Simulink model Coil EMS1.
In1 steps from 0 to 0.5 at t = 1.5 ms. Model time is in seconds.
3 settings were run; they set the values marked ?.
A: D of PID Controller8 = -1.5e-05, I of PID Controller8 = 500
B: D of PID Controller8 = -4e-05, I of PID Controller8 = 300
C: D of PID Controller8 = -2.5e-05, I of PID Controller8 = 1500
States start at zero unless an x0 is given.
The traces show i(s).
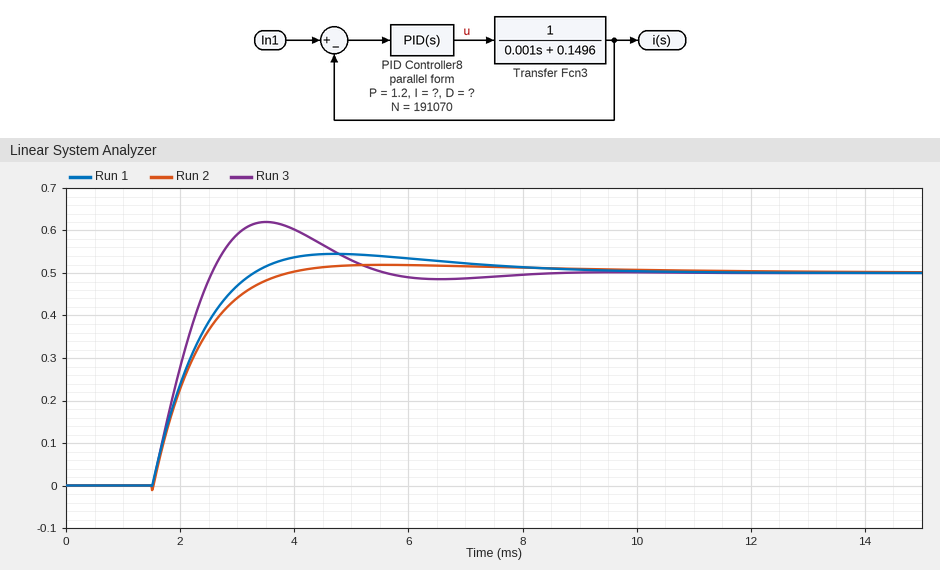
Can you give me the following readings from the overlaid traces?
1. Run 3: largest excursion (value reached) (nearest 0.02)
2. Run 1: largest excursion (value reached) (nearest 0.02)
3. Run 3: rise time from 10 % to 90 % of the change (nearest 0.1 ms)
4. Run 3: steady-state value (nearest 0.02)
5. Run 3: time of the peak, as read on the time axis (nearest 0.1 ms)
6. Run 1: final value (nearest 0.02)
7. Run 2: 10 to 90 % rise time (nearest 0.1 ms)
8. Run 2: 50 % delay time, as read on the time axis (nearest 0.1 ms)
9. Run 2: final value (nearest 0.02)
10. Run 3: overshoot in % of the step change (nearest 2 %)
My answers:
0.62
0.54
0.8 ms
0.50
3.5 ms
0.50
1.5 ms
2.1 ms
0.50
24 %
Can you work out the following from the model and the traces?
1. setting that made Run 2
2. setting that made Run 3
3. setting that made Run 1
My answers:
B
C
A
